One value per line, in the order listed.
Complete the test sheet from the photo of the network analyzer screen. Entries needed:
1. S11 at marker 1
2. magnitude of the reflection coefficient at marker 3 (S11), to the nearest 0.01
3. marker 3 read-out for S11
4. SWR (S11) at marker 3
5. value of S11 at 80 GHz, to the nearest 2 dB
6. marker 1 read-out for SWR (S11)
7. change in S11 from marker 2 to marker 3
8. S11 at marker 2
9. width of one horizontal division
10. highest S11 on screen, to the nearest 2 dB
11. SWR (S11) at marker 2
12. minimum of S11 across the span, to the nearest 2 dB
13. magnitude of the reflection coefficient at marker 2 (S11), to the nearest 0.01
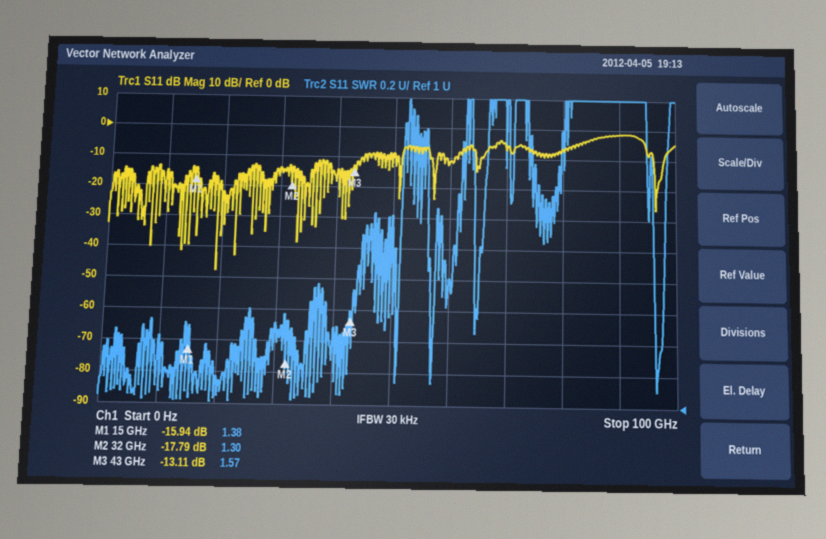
-15.94 dB
0.22
-13.11 dB
1.57
-6 dB
1.38
4.68 dB
-17.79 dB
10 GHz
-2 dB
1.30
-48 dB
0.13
